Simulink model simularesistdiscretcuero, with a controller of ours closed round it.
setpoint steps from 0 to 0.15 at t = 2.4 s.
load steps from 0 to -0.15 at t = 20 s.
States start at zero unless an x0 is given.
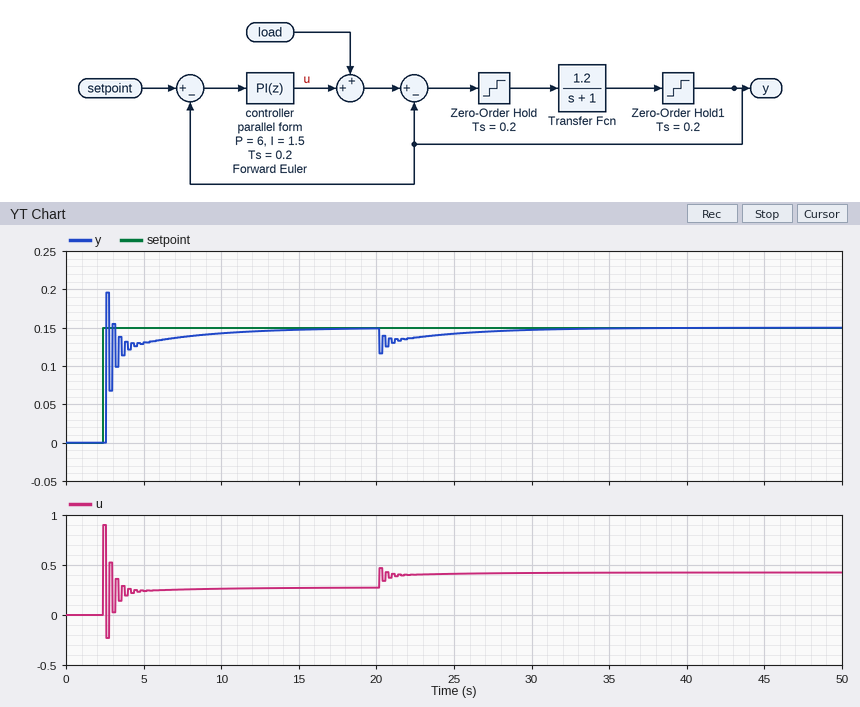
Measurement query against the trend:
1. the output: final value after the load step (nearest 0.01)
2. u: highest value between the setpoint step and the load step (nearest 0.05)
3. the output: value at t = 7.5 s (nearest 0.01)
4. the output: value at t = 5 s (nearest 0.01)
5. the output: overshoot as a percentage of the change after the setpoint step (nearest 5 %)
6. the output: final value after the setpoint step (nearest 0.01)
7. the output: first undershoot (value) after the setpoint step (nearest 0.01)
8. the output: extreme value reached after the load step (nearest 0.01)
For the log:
0.15
0.90
0.14
0.13
30 %
0.15
0.07
0.12
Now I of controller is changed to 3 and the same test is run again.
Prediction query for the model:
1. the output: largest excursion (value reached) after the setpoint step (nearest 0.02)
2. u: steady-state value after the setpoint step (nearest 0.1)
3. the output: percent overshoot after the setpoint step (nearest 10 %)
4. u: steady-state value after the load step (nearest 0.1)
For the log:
0.20
0.3
30 %
0.4
